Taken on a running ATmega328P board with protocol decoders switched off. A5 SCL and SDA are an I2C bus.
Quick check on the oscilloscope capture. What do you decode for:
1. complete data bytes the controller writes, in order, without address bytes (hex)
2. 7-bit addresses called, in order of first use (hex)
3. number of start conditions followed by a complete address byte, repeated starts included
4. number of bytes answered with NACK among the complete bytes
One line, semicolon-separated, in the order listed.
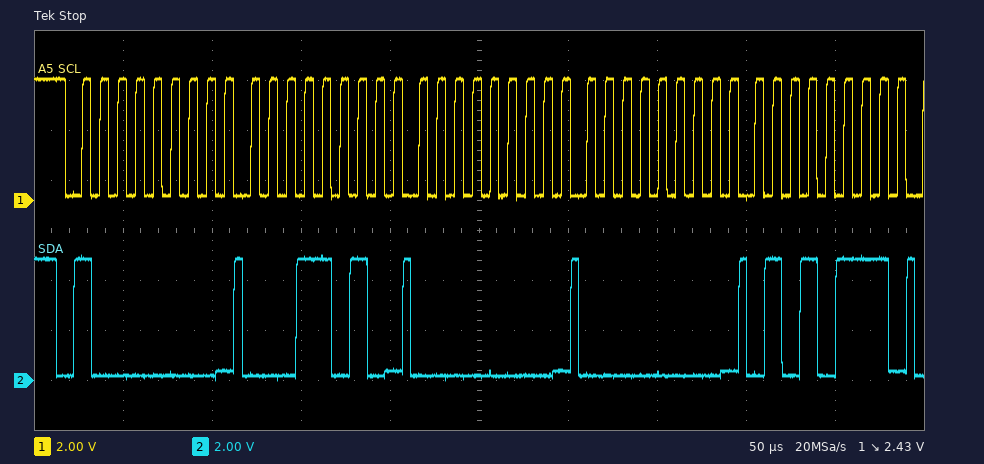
1A 00 00 57; 0x40; 1; 0
